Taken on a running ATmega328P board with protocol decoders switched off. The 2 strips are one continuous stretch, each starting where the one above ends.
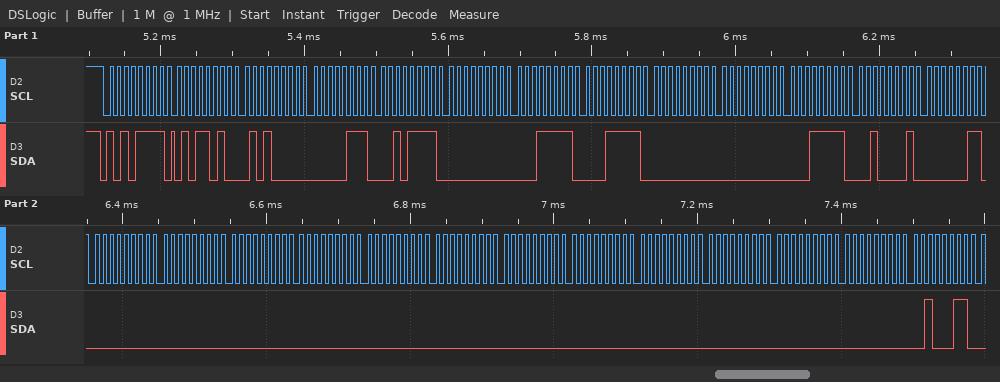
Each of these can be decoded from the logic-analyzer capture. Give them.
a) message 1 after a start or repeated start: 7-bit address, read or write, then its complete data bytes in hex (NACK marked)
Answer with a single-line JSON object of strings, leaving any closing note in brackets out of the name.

{"message 1 after a start or repeated start: 7-bit address, read or write, then its complete data bytes in hex": "0x57 read: 5A 50 07 2F 00 1F 1F 00 00 1F 21 03 00 00 00 00 00 00 00 00 00 00 00 00 23"}
